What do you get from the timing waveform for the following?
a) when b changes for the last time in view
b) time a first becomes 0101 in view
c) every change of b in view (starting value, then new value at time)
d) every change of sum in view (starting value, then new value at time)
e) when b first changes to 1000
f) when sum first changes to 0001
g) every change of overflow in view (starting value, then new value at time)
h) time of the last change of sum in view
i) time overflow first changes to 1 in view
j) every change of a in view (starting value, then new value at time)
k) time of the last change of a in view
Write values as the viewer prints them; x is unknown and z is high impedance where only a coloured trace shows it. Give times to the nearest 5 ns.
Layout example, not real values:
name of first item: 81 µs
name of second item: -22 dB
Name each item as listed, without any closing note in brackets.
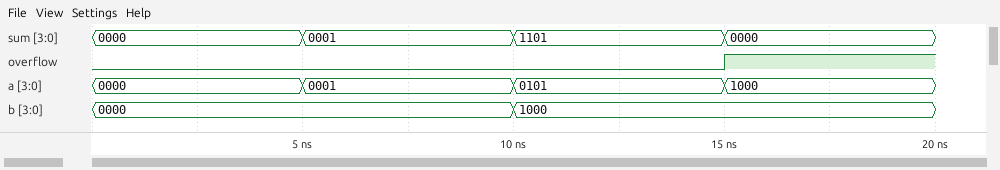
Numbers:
when b changes for the last time in view: 10 ns
time a first becomes 0101 in view: 10 ns
every change of b in view: 0000, 1000 at 10 ns
every change of sum in view: 0000, 0001 at 5 ns, 1101 at 10 ns, 0000 at 15 ns
when b first changes to 1000: 10 ns
when sum first changes to 0001: 5 ns
every change of overflow in view: 0, 1 at 15 ns
time of the last change of sum in view: 15 ns
time overflow first changes to 1 in view: 15 ns
every change of a in view: 0000, 0001 at 5 ns, 0101 at 10 ns, 1000 at 15 ns
time of the last change of a in view: 15 ns
